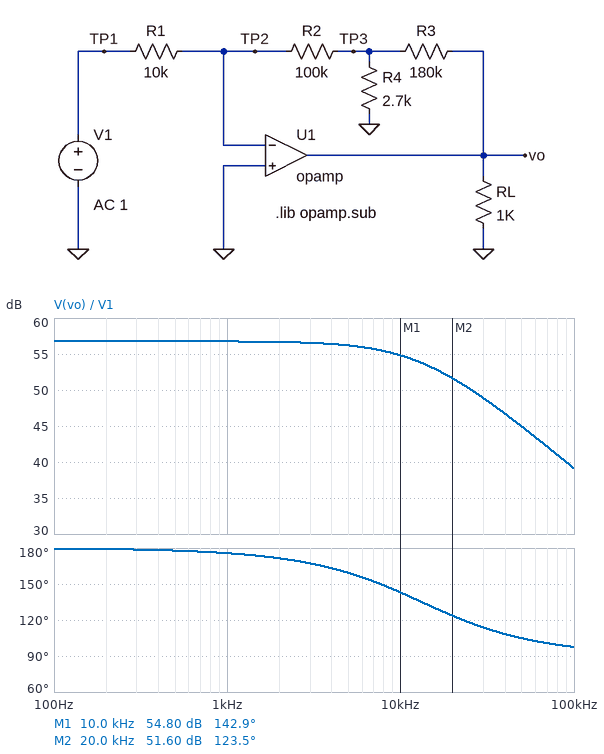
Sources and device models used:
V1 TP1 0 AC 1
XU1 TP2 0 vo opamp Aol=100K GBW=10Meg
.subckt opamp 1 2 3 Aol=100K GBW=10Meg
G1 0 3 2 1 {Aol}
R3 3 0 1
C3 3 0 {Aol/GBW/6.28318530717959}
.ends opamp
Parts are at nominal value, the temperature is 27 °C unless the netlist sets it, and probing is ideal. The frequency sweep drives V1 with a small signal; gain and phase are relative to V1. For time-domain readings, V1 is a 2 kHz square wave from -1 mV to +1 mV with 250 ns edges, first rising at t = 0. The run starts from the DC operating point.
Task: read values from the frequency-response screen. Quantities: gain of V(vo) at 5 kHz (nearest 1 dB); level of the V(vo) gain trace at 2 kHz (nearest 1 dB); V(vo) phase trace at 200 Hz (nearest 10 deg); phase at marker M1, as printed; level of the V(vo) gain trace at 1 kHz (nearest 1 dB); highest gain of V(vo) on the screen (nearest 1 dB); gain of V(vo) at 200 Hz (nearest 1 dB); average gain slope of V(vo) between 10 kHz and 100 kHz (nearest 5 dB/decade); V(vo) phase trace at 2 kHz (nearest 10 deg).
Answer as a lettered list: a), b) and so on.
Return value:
a) 56 dB
b) 57 dB
c) 180 deg
d) 142.9 deg
e) 57 dB
f) 57 dB
g) 57 dB
h) -15 dB/decade
i) 170 deg
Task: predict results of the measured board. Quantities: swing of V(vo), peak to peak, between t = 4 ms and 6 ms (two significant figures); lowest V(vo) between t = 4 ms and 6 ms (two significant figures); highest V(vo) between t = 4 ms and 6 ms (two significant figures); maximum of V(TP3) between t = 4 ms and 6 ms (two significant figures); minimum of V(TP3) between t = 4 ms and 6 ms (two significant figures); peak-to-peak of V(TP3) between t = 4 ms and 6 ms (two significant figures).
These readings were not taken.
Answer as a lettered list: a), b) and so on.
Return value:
a) 1.4 V
b) -690 mV
c) 690 mV
d) 9.9 mV
e) -9.9 mV
f) 20 mV
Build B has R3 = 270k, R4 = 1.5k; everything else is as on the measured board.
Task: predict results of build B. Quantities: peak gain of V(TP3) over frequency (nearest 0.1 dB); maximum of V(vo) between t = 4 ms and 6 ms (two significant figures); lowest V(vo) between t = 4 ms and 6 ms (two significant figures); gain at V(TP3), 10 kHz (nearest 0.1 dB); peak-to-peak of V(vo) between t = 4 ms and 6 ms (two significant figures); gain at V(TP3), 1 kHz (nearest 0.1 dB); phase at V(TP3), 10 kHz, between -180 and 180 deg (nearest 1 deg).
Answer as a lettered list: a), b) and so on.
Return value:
a) 19.8 dB
b) 1.8 V
c) -1.8 V
d) 12.9 dB
e) 3.6 V
f) 19.7 dB
g) 117 deg
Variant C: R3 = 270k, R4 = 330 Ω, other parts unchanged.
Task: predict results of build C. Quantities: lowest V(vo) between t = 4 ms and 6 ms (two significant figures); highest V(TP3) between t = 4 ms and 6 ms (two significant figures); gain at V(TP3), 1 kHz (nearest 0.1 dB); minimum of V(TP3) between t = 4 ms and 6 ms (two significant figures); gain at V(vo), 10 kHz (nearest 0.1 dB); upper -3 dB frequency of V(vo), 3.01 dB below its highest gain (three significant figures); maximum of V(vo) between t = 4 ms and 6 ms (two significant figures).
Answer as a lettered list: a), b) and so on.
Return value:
a) -5.6 V
b) 6.8 mV
c) 17.0 dB
d) -6.8 mV
e) 59.1 dB
f) 1.21 kHz
g) 5.6 V
